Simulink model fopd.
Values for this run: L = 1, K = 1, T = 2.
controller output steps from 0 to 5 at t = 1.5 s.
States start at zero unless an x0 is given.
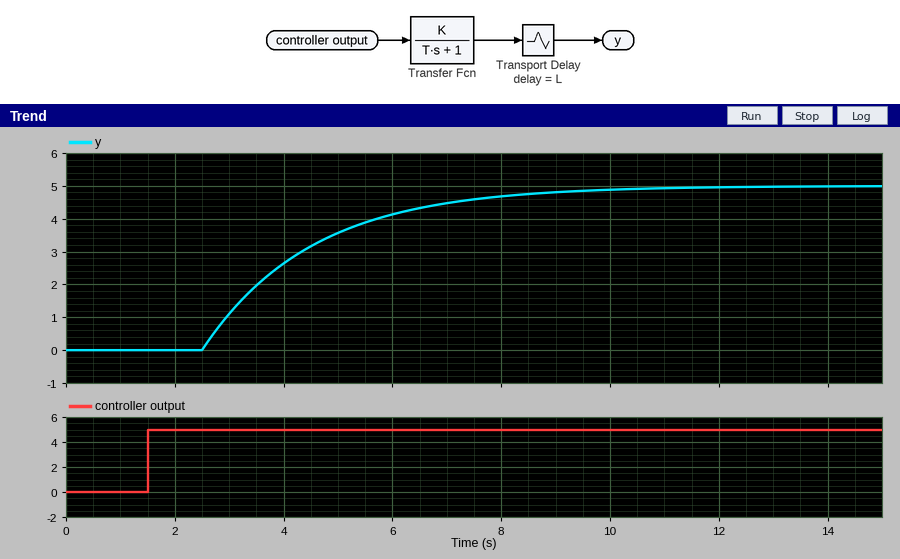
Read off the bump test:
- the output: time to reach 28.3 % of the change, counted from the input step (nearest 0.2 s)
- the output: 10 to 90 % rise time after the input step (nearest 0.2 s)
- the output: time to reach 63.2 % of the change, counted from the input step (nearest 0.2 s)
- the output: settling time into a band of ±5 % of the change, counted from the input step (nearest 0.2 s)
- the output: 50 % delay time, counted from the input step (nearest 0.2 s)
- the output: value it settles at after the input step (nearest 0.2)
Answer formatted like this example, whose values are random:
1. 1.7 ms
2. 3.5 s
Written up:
1. 1.6 s
2. 4.4 s
3. 3.0 s
4. 7.0 s
5. 2.4 s
6. 5.0
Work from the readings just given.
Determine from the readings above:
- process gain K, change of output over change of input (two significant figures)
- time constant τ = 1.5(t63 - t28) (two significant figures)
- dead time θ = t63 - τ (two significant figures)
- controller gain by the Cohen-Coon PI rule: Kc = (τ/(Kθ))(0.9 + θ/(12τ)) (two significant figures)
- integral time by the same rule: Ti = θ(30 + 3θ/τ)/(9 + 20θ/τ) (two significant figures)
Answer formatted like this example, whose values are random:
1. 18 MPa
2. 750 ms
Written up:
1. 1.0
2. 2.1 s
3. 0.90 s
4. 2.2
5. 1.6 s
